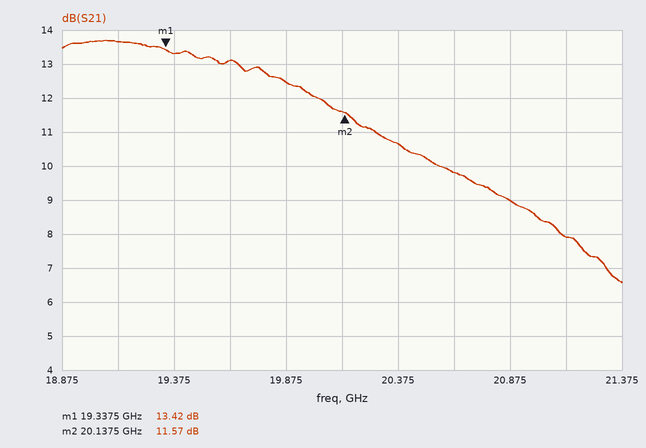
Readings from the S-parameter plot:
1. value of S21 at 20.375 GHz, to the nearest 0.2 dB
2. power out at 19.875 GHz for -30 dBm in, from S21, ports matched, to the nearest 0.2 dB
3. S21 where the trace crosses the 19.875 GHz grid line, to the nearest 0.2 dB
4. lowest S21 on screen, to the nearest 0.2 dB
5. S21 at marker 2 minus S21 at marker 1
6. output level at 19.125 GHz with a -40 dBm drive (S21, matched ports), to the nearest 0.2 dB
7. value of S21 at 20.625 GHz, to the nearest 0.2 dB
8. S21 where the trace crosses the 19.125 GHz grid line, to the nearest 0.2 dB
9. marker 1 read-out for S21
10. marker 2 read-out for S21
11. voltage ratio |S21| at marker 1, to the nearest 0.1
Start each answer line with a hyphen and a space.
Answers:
- 10.6 dB
- -17.6 dBm
- 12.4 dB
- 6.6 dB
- -1.85 dB
- -26.4 dBm
- 9.8 dB
- 13.6 dB
- 13.42 dB
- 11.57 dB
- 4.7
